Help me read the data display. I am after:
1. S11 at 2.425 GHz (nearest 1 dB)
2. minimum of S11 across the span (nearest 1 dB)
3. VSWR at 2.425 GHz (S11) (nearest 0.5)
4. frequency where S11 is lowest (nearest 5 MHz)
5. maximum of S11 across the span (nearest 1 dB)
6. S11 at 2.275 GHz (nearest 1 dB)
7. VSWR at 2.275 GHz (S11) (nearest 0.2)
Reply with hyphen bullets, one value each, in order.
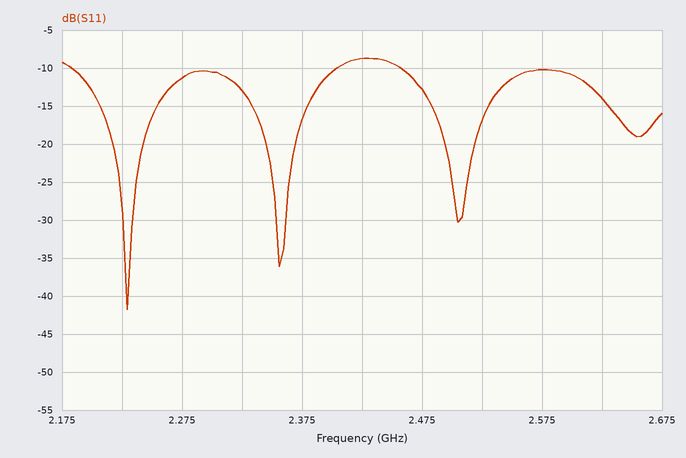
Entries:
- -9 dB
- -42 dB
- 2.0
- 2.230 GHz
- -9 dB
- -11 dB
- 1.8
